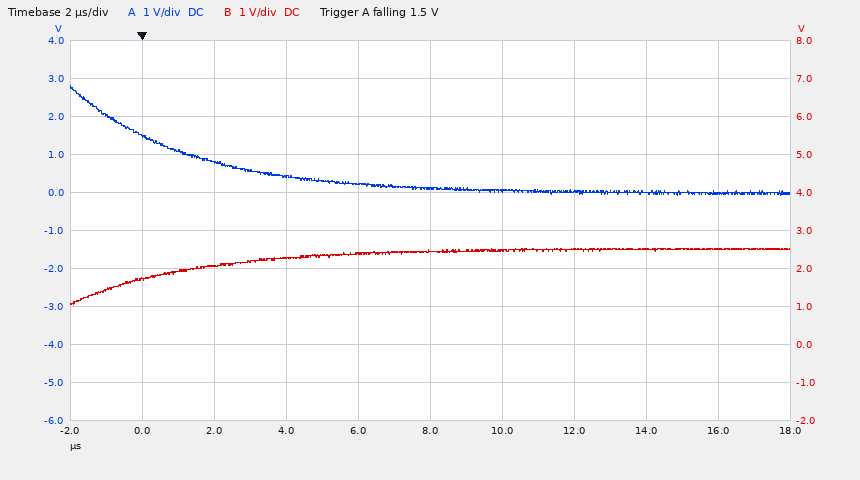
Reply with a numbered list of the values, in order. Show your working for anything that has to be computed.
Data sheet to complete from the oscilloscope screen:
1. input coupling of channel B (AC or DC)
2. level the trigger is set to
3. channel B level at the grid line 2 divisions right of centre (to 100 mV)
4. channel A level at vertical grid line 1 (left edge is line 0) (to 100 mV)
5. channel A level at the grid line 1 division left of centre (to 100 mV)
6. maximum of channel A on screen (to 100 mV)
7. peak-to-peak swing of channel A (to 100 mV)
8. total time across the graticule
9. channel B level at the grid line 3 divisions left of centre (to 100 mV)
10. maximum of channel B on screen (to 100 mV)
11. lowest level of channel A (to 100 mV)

1. DC
2. 1.5 V
3. 2.5 V
4. 1.5 V
5. 200 mV
6. 2.8 V
7. 2.8 V − (-100 mV) = 2.9 V
8. 20 µs
9. 2.1 V
10. 2.5 V
11. -100 mV
